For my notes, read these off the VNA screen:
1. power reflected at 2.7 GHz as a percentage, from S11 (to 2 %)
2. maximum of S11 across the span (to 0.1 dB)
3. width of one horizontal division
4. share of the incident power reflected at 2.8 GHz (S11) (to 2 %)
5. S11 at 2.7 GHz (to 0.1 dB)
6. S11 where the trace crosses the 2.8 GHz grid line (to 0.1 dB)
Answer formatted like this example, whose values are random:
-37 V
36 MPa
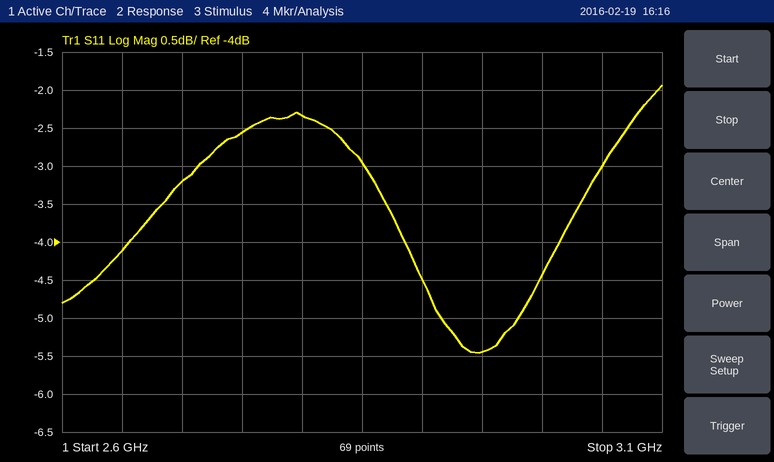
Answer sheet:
48 %
-1.9 dB
50 MHz
58 %
-3.2 dB
-2.3 dB
